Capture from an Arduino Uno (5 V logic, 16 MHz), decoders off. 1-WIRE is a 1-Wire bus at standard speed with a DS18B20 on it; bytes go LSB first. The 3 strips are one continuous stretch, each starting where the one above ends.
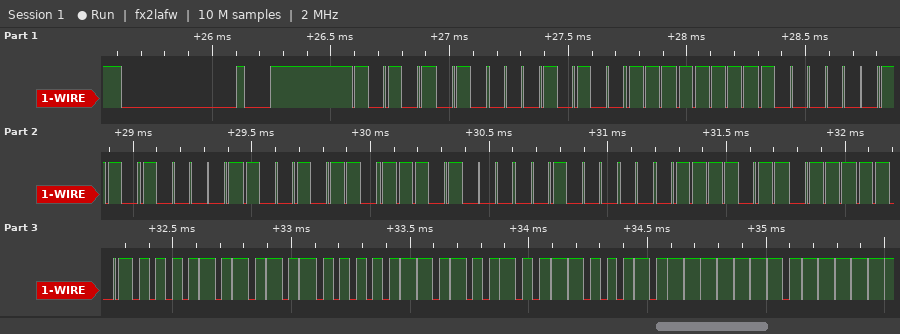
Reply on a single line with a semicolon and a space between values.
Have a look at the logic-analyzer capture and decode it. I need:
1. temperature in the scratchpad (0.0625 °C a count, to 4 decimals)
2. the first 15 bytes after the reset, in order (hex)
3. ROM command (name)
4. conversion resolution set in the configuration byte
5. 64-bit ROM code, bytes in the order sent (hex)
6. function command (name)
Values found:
85.0000 °C; 55 28 FF 81 85 69 17 04 DE BE 50 05 4B 46 7F; Match ROM; 12 bits; 28 FF 81 85 69 17 04 DE; Read Scratchpad
